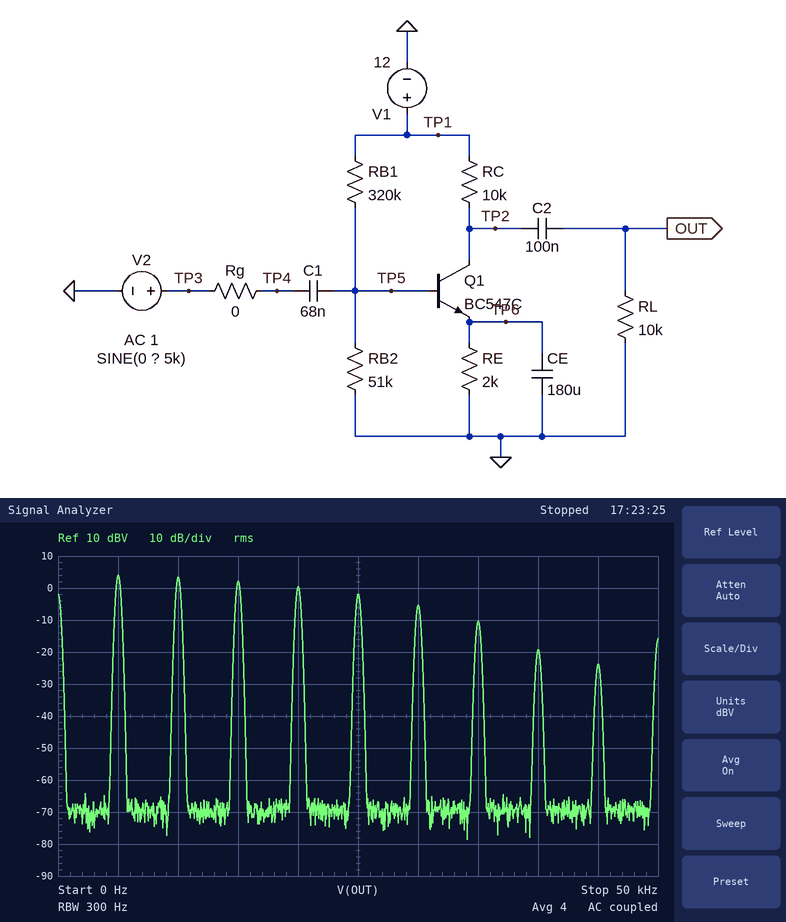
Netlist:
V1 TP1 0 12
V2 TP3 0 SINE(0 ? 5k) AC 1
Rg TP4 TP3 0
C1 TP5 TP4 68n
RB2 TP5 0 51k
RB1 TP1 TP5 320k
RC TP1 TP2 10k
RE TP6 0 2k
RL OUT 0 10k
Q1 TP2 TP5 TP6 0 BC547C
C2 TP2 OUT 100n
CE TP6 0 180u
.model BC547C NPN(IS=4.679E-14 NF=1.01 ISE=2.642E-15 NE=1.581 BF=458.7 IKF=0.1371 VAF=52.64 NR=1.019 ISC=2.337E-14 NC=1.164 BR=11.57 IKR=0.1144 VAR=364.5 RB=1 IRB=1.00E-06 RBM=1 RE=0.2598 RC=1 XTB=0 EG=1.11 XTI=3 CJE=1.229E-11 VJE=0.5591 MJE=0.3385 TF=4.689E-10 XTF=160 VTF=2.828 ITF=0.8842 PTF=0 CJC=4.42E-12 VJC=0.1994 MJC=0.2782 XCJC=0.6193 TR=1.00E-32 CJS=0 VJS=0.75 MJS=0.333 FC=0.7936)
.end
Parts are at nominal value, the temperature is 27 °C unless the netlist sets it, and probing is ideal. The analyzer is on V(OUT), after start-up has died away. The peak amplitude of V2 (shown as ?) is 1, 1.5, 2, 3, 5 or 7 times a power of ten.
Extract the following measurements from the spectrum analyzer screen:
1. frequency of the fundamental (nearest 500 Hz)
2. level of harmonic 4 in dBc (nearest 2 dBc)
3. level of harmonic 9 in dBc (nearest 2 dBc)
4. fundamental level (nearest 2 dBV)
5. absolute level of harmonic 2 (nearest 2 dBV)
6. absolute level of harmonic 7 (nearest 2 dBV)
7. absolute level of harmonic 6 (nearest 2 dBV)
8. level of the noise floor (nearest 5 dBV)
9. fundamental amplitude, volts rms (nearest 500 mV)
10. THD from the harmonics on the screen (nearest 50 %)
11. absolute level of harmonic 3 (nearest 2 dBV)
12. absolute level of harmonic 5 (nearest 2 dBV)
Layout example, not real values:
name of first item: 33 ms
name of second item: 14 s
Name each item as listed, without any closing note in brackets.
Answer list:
frequency of the fundamental: 5.0 kHz
level of harmonic 4 in dBc: -4 dBc
level of harmonic 9 in dBc: -28 dBc
fundamental level: 4 dBV
absolute level of harmonic 2: 4 dBV
absolute level of harmonic 7: -10 dBV
absolute level of harmonic 6: -6 dBV
level of the noise floor: -70 dBV
fundamental amplitude, volts rms: 1.5 V
THD from the harmonics on the screen: 150 %
absolute level of harmonic 3: 2 dBV
absolute level of harmonic 5: -2 dBV
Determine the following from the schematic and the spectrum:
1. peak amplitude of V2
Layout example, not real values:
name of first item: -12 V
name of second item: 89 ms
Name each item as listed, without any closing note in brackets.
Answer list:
peak amplitude of V2: 1 V
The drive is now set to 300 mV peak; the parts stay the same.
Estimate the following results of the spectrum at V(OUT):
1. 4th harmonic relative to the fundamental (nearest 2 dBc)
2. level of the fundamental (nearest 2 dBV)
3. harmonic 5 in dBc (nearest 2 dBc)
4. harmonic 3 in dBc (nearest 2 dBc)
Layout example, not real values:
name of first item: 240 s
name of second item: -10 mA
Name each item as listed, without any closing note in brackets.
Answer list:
4th harmonic relative to the fundamental: -8 dBc
level of the fundamental: 6 dBV
harmonic 5 in dBc: -16 dBc
harmonic 3 in dBc: -4 dBc
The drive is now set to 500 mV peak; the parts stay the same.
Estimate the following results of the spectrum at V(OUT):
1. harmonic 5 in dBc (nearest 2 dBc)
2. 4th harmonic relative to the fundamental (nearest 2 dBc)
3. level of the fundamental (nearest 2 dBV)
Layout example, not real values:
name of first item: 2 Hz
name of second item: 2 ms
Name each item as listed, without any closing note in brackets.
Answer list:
harmonic 5 in dBc: -10 dBc
4th harmonic relative to the fundamental: -6 dBc
level of the fundamental: 6 dBV
